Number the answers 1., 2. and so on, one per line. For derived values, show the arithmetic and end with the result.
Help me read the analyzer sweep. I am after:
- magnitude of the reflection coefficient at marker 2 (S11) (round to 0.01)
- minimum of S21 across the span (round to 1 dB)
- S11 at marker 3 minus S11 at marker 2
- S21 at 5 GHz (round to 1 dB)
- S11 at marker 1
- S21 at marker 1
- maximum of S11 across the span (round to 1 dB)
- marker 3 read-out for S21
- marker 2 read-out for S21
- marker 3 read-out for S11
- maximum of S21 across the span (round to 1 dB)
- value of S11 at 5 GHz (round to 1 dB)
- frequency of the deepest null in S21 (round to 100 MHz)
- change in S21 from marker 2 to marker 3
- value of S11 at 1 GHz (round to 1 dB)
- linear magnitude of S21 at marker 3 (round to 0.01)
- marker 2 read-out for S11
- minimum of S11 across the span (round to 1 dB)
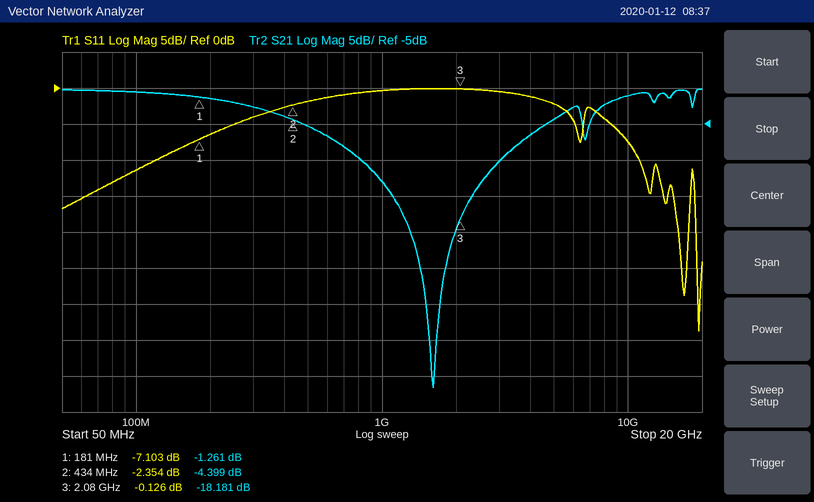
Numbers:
1. 10^(-2.354/20) ≈ 0.76
2. -42 dB
3. -0.126 − (-2.354) = 2.228 dB
4. -4 dB
5. -7.103 dB
6. -1.261 dB
7. 0 dB
8. -18.181 dB
9. -4.399 dB
10. -0.126 dB
11. 0 dB
12. -2 dB
13. 1.6 GHz
14. -18.181 − (-4.399) = -13.782 dB
15. 0 dB
16. 10^(-18.181/20) ≈ 0.12
17. -2.354 dB
18. -34 dB
